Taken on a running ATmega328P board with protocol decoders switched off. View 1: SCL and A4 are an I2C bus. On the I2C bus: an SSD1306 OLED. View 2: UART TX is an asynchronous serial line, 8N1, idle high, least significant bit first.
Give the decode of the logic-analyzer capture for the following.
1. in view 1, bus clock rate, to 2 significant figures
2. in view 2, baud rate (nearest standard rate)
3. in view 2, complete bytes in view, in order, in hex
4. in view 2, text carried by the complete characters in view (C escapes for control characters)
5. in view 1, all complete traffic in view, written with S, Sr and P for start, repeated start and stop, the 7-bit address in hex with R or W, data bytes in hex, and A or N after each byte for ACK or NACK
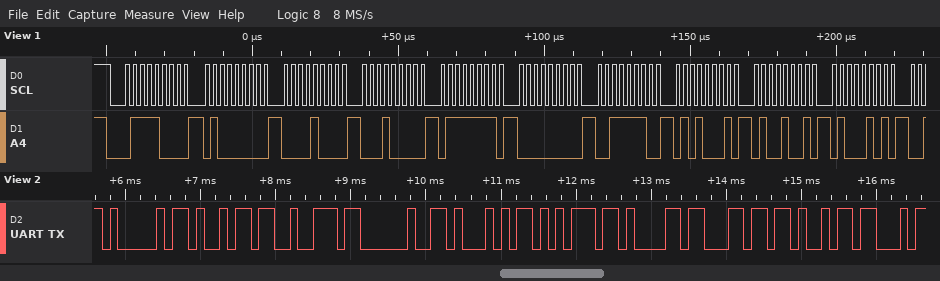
400 kHz
9600 baud
41 69 72 20 51 75 61 6C 69
"Air Quali"
S 3CW A 40 A 08 A 10 A 7F A 00 A 3E A 51 A 49 A 45 A
